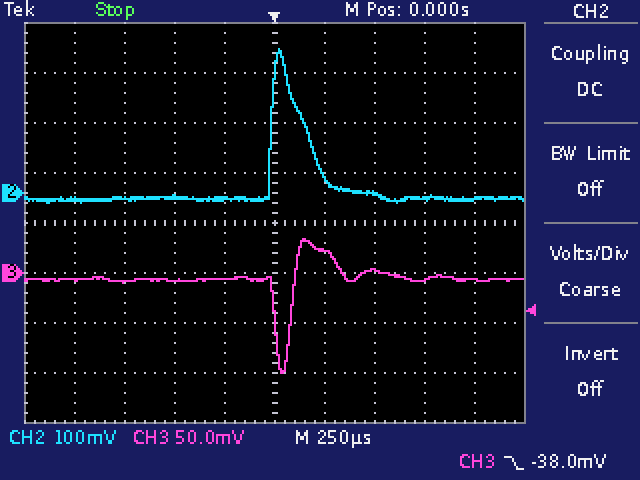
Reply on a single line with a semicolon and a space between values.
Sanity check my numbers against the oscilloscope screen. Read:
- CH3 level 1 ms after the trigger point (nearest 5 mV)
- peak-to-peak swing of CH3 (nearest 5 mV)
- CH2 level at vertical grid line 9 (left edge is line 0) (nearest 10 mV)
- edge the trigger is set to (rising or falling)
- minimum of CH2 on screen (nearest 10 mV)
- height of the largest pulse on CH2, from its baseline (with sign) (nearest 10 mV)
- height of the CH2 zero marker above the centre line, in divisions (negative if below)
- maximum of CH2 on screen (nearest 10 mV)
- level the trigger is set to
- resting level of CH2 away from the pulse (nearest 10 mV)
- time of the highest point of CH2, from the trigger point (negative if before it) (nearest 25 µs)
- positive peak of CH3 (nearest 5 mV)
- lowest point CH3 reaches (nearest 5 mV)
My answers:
-5 mV; 135 mV; -10 mV; falling; -20 mV; +300 mV; +0.6 div; 290 mV; -38.0 mV; -10 mV; +25 µs; 35 mV; -100 mV
